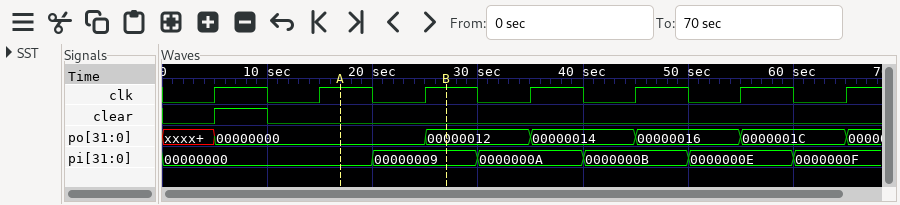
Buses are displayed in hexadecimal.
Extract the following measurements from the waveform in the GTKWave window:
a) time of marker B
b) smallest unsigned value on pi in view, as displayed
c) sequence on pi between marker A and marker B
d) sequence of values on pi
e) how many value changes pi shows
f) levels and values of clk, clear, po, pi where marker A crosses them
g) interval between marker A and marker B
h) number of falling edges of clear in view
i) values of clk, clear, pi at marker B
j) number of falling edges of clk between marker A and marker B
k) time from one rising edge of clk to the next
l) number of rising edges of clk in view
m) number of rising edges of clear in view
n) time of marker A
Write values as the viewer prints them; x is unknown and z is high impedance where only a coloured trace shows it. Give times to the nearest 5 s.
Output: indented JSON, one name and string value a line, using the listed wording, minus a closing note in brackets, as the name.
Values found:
{
  "time of marker B": "25 s",
  "smallest unsigned value on pi in view, as displayed": "00000000",
  "sequence on pi between marker A and marker B": "00000000, 00000009",
  "sequence of values on pi": "00000000, 00000009, 0000000A, 0000000B, 0000000E, 0000000F",
  "how many value changes pi shows": "5",
  "levels and values of clk, clear, po, pi where marker A crosses them": "clk=1, clear=0, po=00000000, pi=00000000",
  "interval between marker A and marker B": "10 s",
  "number of falling edges of clear in view": "1",
  "values of clk, clear, pi at marker B": "clk=1, clear=0, pi=00000009",
  "number of falling edges of clk between marker A and marker B": "1",
  "time from one rising edge of clk to the next": "10 s",
  "number of rising edges of clk in view": "7",
  "number of rising edges of clear in view": "1",
  "time of marker A": "15 s"
}
